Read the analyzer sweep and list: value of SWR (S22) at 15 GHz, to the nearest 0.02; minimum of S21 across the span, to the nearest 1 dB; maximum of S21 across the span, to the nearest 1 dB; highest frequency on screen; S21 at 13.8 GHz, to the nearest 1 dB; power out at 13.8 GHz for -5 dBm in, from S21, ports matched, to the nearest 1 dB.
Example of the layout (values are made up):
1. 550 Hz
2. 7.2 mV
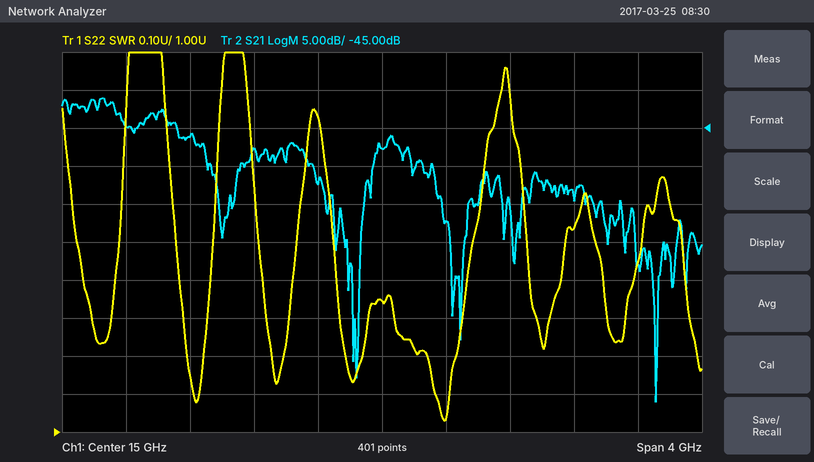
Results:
1. 1.34
2. -81 dB
3. -41 dB
4. 17 GHz
5. -46 dB
6. -51 dBm
